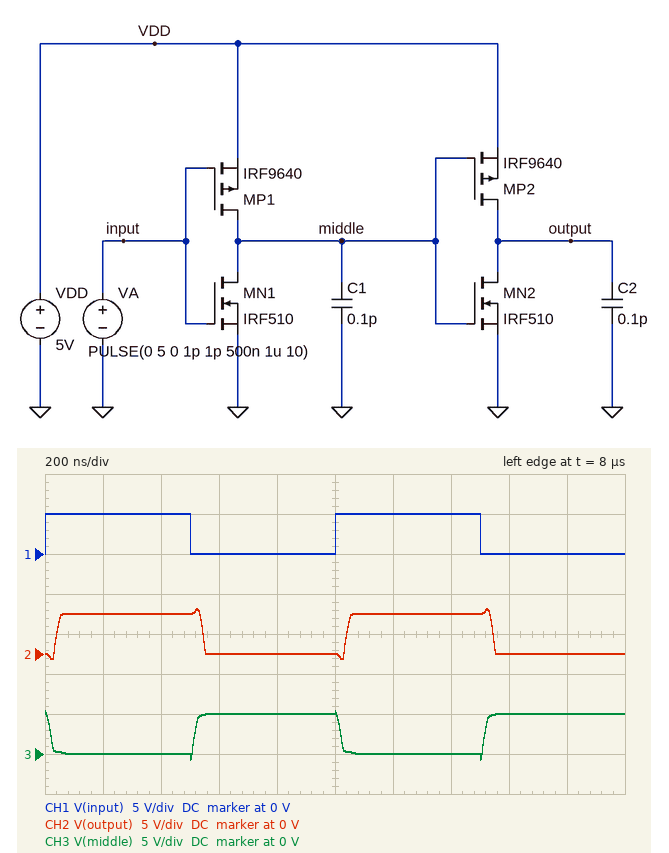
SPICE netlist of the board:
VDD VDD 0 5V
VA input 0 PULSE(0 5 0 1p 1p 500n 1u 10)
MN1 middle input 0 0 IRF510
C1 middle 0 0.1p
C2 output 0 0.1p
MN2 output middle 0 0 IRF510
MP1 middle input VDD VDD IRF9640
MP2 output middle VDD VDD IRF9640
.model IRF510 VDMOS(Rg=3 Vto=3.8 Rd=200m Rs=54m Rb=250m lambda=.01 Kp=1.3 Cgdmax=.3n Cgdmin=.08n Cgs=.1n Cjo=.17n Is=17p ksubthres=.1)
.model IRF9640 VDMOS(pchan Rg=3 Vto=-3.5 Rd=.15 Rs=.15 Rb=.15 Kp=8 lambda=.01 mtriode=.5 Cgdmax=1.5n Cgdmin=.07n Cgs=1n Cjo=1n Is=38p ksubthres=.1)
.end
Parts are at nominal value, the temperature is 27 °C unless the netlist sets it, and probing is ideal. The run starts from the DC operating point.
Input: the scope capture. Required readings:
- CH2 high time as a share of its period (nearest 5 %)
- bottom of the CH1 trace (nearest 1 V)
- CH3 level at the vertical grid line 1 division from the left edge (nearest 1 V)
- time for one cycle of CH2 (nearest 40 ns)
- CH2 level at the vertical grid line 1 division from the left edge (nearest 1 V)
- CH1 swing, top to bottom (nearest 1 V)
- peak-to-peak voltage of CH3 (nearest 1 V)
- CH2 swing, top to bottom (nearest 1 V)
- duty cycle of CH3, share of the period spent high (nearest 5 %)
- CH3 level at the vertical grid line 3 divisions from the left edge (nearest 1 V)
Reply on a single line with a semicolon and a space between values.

50 %; 0 V; 0 V; 1.00 µs; 5 V; 5 V; 6 V; 6 V; 50 %; 5 V
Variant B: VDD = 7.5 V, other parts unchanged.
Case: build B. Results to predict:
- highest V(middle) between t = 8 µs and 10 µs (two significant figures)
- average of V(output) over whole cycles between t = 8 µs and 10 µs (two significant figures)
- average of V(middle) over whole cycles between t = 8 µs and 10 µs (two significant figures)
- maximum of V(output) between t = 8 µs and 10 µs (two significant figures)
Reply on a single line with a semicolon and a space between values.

7.8 V; 3.6 V; 3.9 V; 7.7 V
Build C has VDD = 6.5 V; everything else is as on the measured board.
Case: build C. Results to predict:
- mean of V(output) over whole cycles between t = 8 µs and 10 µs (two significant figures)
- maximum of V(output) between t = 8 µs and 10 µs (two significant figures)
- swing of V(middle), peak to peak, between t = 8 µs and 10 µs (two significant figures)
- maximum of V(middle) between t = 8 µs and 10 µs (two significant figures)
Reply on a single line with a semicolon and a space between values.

3.1 V; 6.7 V; 7.5 V; 6.8 V
